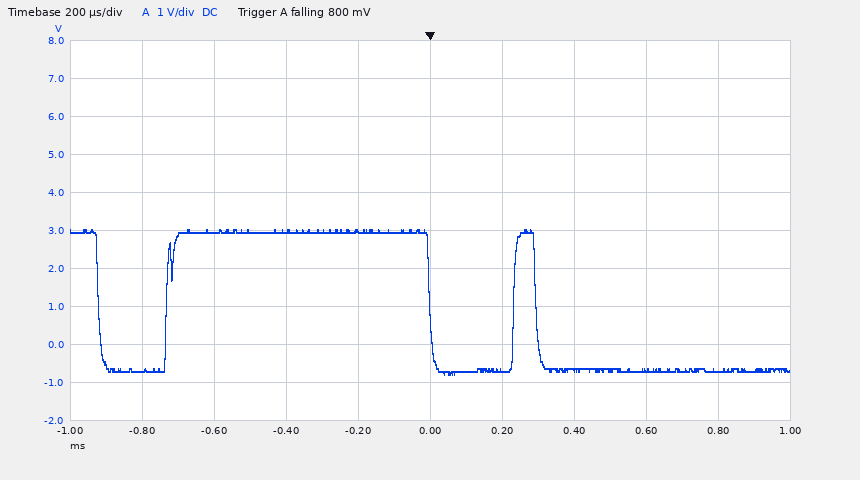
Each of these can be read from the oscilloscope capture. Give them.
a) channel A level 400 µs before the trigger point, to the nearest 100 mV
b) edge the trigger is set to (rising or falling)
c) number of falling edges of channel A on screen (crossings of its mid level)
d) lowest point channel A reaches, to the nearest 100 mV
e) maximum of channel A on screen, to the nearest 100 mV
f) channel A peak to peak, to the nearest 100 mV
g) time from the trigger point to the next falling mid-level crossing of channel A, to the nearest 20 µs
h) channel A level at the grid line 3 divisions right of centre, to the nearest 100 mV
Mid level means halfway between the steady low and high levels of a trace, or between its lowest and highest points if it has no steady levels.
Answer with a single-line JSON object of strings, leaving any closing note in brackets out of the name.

{"channel A level 400 µs before the trigger point, to the nearest 100 mV": "3.0 V", "edge the trigger is set to": "falling", "number of falling edges of channel A on screen": "3", "lowest point channel A reaches, to the nearest 100 mV": "-800 mV", "maximum of channel A on screen, to the nearest 100 mV": "3.0 V", "channel A peak to peak, to the nearest 100 mV": "3.8 V", "time from the trigger point to the next falling mid-level crossing of channel A, to the nearest 20 µs": "300 µs", "channel A level at the grid line 3 divisions right of centre, to the nearest 100 mV": "-700 mV"}
